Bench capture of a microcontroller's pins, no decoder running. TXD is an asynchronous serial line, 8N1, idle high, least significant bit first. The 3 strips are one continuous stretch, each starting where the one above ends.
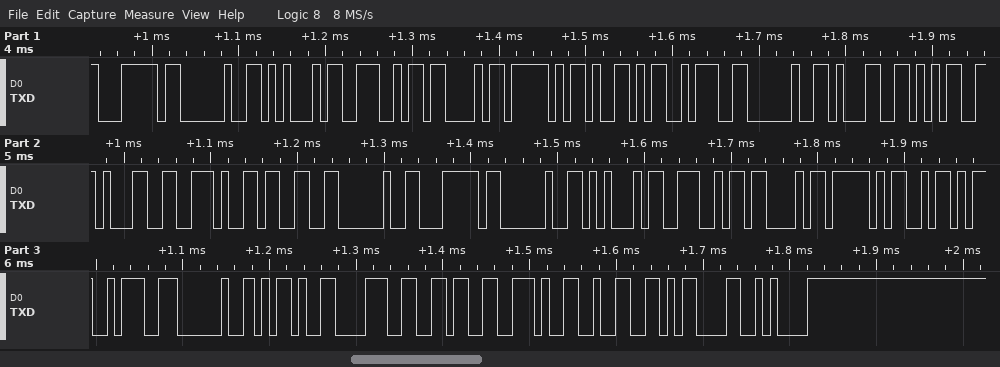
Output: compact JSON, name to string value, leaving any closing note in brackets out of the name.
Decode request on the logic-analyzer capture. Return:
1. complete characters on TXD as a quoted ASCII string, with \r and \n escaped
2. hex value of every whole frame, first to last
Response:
{"complete characters on TXD as a quoted ASCII string, with \\r and \\n escaped": "\"| ENC_Y: 151.3 | ENC_Z: -86.2\\r\\n\"", "hex value of every whole frame, first to last": "7C 20 45 4E 43 5F 59 3A 20 31 35 31 2E 33 20 7C 20 45 4E 43 5F 5A 3A 20 2D 38 36 2E 32 0D 0A"}
